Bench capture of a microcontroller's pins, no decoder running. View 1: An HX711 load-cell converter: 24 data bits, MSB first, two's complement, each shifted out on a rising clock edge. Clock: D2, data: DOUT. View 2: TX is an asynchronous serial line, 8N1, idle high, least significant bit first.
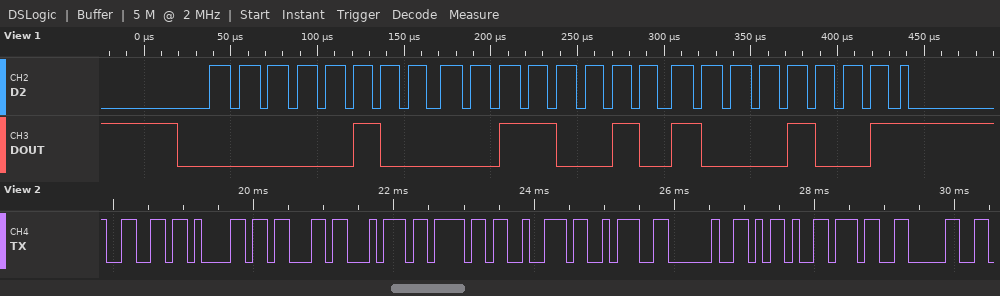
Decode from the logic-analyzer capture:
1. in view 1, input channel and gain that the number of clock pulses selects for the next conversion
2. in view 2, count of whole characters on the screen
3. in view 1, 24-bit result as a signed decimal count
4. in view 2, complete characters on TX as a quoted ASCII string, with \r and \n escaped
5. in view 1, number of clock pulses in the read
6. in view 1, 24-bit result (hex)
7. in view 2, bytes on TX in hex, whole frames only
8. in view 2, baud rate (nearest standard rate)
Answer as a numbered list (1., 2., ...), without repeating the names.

1. channel A, gain 128
2. 11
3. 275081
4. "factor: -70"
5. 25
6. 0x043289
7. 66 61 63 74 6F 72 3A 20 2D 37 30
8. 9600 baud
